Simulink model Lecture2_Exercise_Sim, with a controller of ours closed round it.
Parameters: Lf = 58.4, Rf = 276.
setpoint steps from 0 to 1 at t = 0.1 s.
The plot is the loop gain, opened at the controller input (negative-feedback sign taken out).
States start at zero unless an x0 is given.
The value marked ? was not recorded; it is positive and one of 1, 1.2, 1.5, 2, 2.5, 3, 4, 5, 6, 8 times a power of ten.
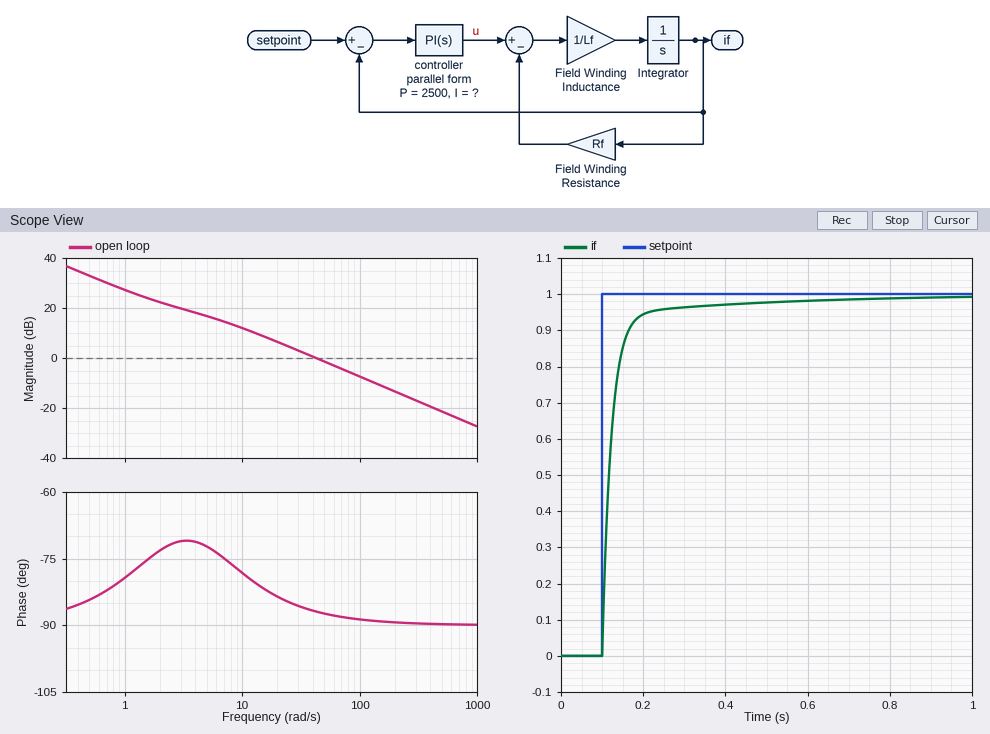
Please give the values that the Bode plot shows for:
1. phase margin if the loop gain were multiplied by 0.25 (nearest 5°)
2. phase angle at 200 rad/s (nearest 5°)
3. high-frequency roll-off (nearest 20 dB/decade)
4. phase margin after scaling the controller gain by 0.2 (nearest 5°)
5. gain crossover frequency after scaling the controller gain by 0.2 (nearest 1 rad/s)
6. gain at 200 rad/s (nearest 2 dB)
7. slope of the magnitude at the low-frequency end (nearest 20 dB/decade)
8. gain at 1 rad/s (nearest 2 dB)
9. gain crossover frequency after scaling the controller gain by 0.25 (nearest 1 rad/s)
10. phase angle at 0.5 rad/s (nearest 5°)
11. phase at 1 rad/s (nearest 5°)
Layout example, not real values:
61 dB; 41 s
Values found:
100°; -90°; -20 dB/decade; 105°; 8 rad/s; -14 dB; -20 dB/decade; 28 dB; 10 rad/s; -85°; -80°
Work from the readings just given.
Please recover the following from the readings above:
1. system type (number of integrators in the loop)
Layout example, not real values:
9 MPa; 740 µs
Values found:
1
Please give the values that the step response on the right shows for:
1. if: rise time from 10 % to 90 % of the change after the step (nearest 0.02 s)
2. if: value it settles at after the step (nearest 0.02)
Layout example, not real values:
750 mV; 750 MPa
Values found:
0.06 s; 1.00
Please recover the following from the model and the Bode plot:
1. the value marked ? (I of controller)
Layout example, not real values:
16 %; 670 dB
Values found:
6000
